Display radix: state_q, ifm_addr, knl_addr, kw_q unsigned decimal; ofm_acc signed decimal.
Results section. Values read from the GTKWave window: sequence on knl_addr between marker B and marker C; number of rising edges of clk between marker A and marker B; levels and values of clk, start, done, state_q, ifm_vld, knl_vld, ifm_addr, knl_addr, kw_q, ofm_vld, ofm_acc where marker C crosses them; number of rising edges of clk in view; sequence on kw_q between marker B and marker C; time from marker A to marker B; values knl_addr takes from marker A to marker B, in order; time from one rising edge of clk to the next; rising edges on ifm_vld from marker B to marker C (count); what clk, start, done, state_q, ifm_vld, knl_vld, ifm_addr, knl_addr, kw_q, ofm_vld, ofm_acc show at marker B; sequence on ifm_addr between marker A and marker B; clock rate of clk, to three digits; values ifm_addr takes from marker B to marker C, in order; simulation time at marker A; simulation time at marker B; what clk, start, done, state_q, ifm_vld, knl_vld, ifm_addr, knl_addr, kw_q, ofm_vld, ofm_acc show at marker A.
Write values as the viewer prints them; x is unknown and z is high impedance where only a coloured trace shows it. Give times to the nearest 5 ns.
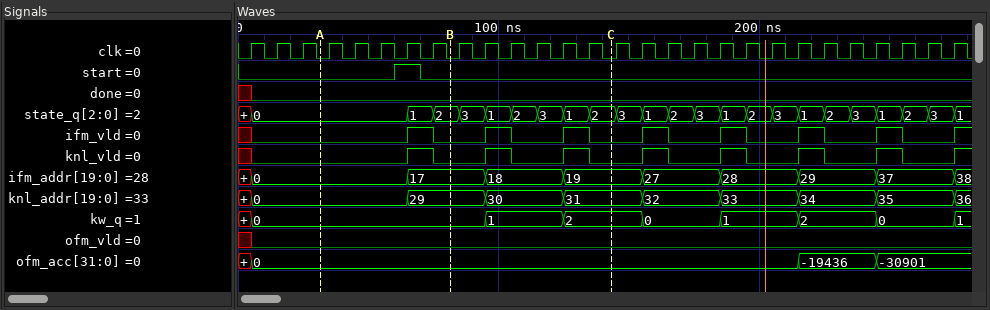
29, 30, 31
5
clk=0, start=0, done=0, state_q=2, ifm_vld=0, knl_vld=0, ifm_addr=19, knl_addr=31, kw_q=2, ofm_vld=0, ofm_acc=0
28
0, 1, 2
50 ns
0, 29
10 ns
2
clk=0, start=0, done=0, state_q=2, ifm_vld=0, knl_vld=0, ifm_addr=17, knl_addr=29, kw_q=0, ofm_vld=0, ofm_acc=0
0, 17
100 MHz
17, 18, 19
30 ns
80 ns
clk=0, start=0, done=0, state_q=0, ifm_vld=0, knl_vld=0, ifm_addr=0, knl_addr=0, kw_q=0, ofm_vld=0, ofm_acc=0
